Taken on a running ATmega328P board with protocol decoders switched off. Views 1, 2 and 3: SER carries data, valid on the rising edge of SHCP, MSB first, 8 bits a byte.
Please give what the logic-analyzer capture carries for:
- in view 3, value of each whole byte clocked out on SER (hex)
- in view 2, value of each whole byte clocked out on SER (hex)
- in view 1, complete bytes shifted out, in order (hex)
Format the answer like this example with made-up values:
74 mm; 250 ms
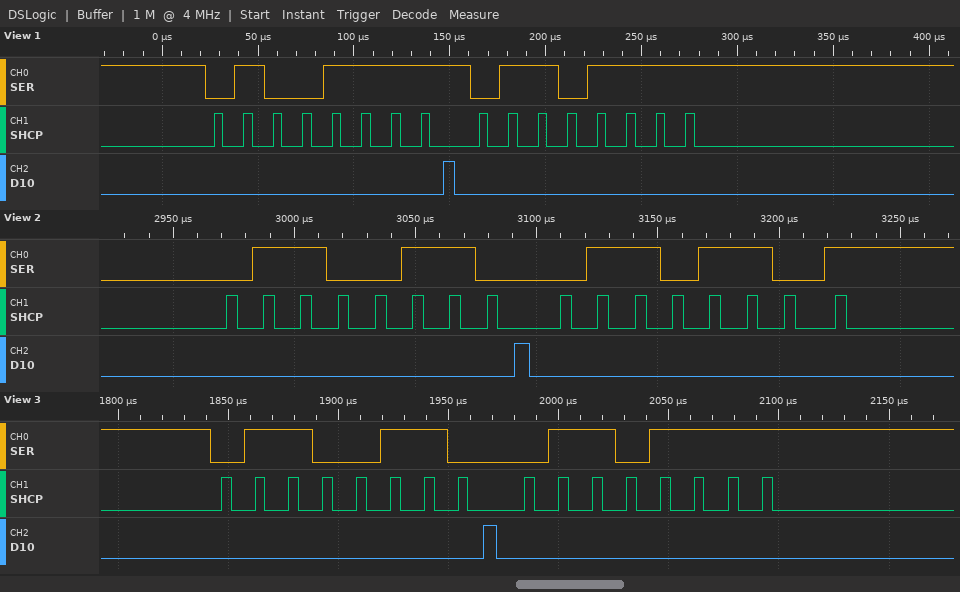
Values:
66 6F; 66 6D; 4F 6F
